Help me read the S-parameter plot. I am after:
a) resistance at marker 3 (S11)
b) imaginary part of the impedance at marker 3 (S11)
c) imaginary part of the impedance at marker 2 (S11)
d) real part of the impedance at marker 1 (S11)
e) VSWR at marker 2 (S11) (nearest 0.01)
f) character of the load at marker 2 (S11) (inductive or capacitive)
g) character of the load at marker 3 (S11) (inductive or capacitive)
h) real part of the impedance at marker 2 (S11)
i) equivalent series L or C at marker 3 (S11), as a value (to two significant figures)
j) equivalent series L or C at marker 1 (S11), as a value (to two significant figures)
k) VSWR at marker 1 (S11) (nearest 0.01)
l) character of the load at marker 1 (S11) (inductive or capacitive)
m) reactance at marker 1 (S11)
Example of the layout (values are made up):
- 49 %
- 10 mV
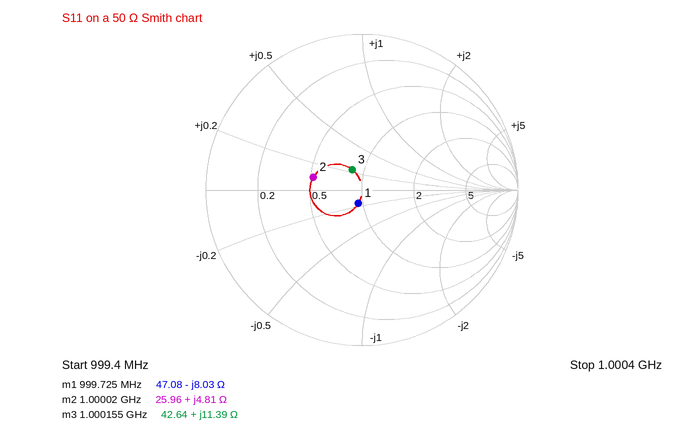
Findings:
- 42.64 Ω
- +11.39 Ω
- +4.81 Ω
- 47.08 Ω
- 1.95
- inductive
- inductive
- 25.96 Ω
- 1.8 nH
- 20 pF
- 1.19
- capacitive
- -8.03 Ω
